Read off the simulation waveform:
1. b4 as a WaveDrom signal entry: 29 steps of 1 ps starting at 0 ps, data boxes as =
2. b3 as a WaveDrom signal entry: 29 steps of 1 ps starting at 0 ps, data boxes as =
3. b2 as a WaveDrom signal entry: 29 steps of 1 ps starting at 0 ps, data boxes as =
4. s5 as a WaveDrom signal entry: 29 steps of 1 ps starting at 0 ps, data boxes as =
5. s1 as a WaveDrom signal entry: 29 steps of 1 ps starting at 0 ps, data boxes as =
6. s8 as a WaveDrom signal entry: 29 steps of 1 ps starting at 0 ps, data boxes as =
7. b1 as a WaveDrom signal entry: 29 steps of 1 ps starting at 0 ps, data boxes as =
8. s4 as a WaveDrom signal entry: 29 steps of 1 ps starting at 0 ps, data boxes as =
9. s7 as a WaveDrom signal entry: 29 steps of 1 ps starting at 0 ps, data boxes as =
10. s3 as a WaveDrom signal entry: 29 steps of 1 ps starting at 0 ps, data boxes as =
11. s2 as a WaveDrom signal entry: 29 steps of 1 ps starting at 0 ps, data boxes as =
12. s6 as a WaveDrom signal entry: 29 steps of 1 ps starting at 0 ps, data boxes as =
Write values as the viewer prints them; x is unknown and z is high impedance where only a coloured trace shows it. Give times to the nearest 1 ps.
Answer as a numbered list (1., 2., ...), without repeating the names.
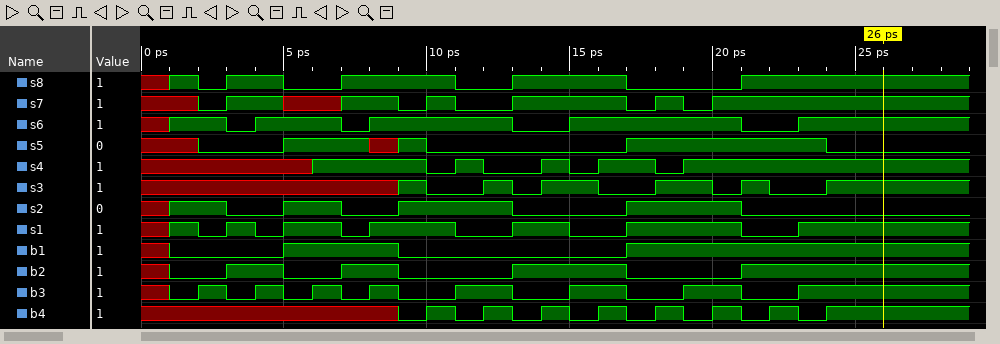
1. {name: 'b4', wave: 'x........0101010101010101....'}
2. {name: 'b3', wave: 'x010101010.1.0.1.0.1.0.1.....'}
3. {name: 'b2', wave: 'x0.1.0.1.0...1...0...1.......'}
4. {name: 's5', wave: 'x.0..1..x10......1......0....'}
5. {name: 's1', wave: 'x10101.01..0.1.0.1...0.1.....'}
6. {name: 's8', wave: 'x101.0.1...0.1...0...1.......'}
7. {name: 'b1', wave: 'x0...1...0.......1...........'}
8. {name: 's4', wave: 'x.....1...010.101.01.........'}
9. {name: 's7', wave: 'x.01.x.1.010.1...0101........'}
10. {name: 's3', wave: 'x........10.101.0.1.010.1....'}
11. {name: 's2', wave: 'x1.0.1.0.1...0...1...0.......'}
12. {name: 's6', wave: 'x1.01..01....0.1.....0.1.....'}
